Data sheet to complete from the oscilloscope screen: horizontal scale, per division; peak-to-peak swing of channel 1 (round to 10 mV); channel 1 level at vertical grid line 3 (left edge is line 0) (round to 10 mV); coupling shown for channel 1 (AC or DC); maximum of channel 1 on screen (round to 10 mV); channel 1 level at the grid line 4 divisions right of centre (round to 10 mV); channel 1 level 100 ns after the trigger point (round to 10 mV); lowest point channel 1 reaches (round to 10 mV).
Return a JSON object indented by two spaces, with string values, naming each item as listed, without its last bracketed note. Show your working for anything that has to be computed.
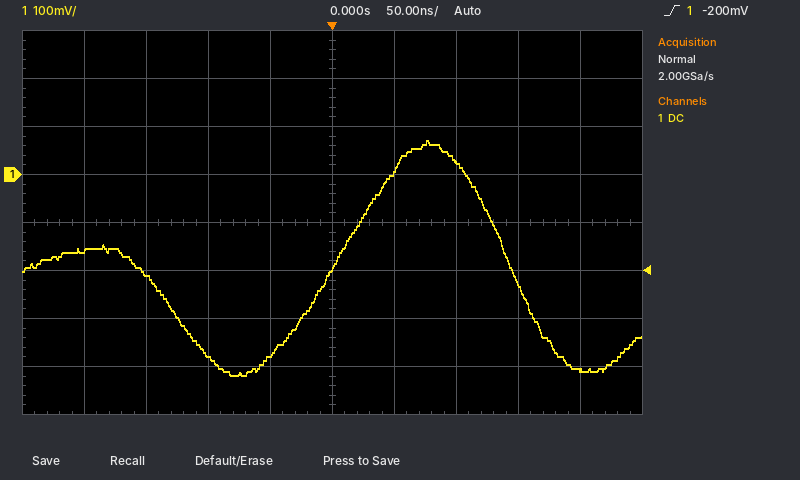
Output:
{
  "horizontal scale, per division": "50 ns",
  "peak-to-peak swing of channel 1": "70 mV − (-420 mV) = 490 mV",
  "channel 1 level at vertical grid line 3 (left edge is line 0)": "-380 mV",
  "coupling shown for channel 1": "DC",
  "maximum of channel 1 on screen": "70 mV",
  "channel 1 level at the grid line 4 divisions right of centre": "-410 mV",
  "channel 1 level 100 ns after the trigger point": "30 mV",
  "lowest point channel 1 reaches": "-420 mV"
}
